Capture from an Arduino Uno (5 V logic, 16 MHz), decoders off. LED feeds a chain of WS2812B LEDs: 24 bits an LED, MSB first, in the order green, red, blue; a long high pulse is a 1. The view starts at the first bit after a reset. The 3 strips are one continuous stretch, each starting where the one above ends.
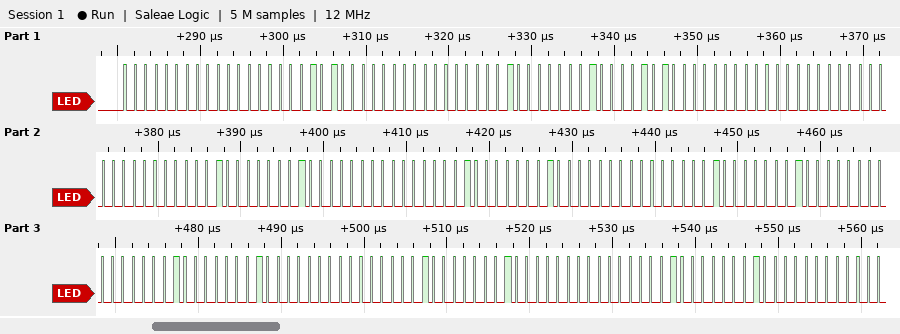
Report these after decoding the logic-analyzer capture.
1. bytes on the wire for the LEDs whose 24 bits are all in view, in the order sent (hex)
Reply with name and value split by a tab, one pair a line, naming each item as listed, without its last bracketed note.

bytes on the wire for the LEDs whose 24 bits are all in view, in the order sent	00 00 28 00 04 04 28 00 00 00 04 04 00 04 04 00 04 04 00 04 04 00 04 04 00 04 04
